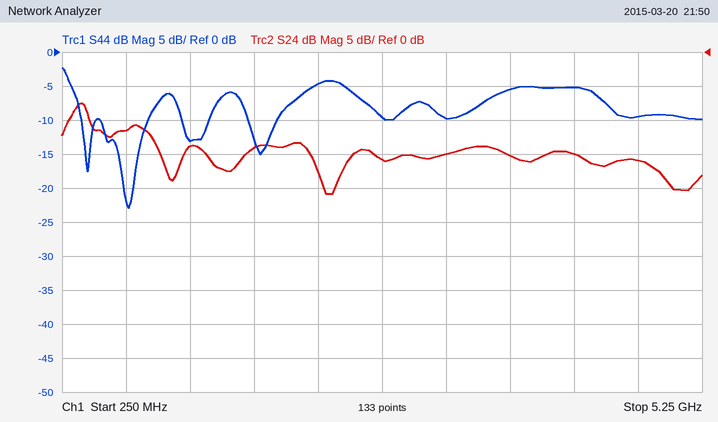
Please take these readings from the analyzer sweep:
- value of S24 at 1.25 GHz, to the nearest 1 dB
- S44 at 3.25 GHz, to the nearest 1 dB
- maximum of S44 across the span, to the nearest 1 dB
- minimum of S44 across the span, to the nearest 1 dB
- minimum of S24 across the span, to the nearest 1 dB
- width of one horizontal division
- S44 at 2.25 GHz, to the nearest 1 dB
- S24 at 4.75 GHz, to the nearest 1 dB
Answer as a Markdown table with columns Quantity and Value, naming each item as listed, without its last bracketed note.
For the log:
| Quantity | Value |
|---|---|
| value of S24 at 1.25 GHz, to the nearest 1 dB | -14 dB |
| S44 at 3.25 GHz, to the nearest 1 dB | -10 dB |
| maximum of S44 across the span, to the nearest 1 dB | -2 dB |
| minimum of S44 across the span, to the nearest 1 dB | -23 dB |
| minimum of S24 across the span, to the nearest 1 dB | -21 dB |
| width of one horizontal division | 500 MHz |
| S44 at 2.25 GHz, to the nearest 1 dB | -5 dB |
| S24 at 4.75 GHz, to the nearest 1 dB | -16 dB |
